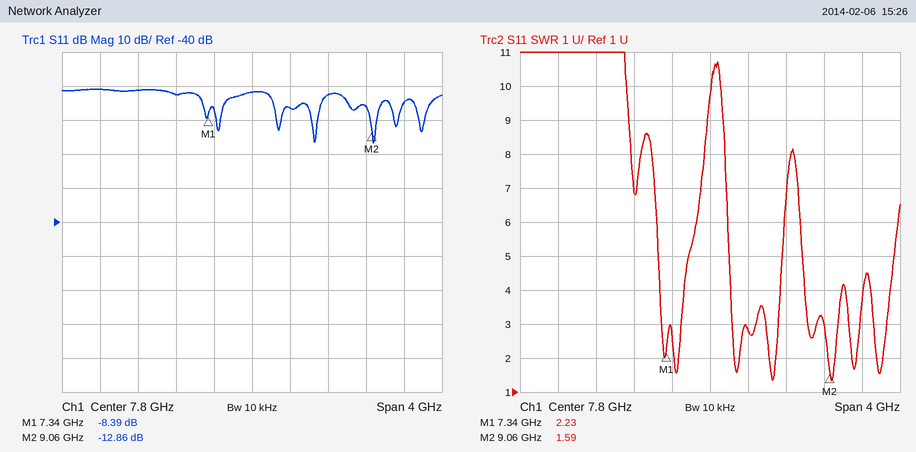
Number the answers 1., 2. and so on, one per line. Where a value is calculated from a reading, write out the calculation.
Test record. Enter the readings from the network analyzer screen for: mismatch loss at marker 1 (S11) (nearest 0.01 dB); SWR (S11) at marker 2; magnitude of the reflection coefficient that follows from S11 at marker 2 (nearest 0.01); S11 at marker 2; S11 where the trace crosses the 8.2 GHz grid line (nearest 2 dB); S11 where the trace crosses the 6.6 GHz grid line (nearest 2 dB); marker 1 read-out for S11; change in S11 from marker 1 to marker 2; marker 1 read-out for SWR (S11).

1. −10 log10(1 − 10^(-8.39/10)) ≈ 0.68 dB
2. 1.59
3. 10^(-12.86/20) ≈ 0.23
4. -12.86 dB
5. -6 dB
6. -2 dB
7. -8.39 dB
8. -12.86 − (-8.39) = -4.47 dB
9. 2.23
